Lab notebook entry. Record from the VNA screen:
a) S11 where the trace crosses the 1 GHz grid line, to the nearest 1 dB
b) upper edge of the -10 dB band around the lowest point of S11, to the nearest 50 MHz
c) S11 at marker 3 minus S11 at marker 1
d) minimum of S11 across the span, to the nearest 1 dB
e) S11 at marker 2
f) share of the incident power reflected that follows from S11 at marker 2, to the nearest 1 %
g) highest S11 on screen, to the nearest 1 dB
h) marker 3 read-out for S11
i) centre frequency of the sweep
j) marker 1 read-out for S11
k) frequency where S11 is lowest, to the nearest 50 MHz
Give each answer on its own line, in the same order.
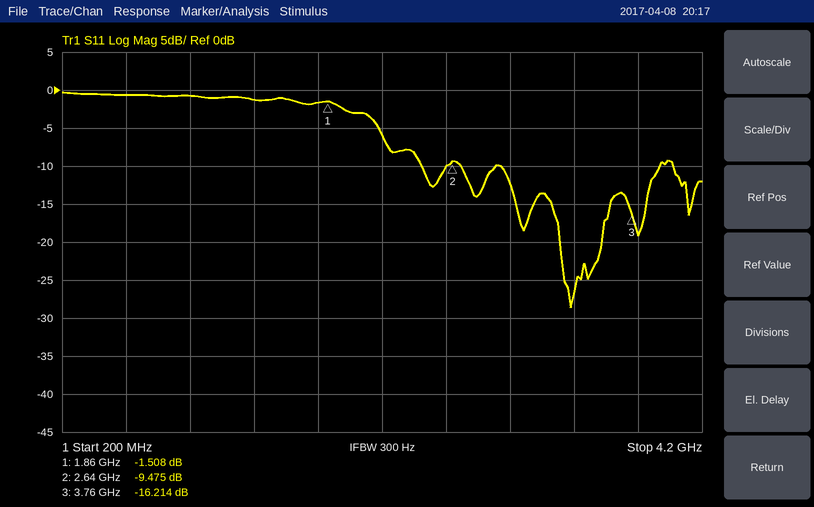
-1 dB
3.95 GHz
-14.706 dB
-29 dB
-9.475 dB
11 %
0 dB
-16.214 dB
2.2 GHz
-1.508 dB
3.40 GHz
